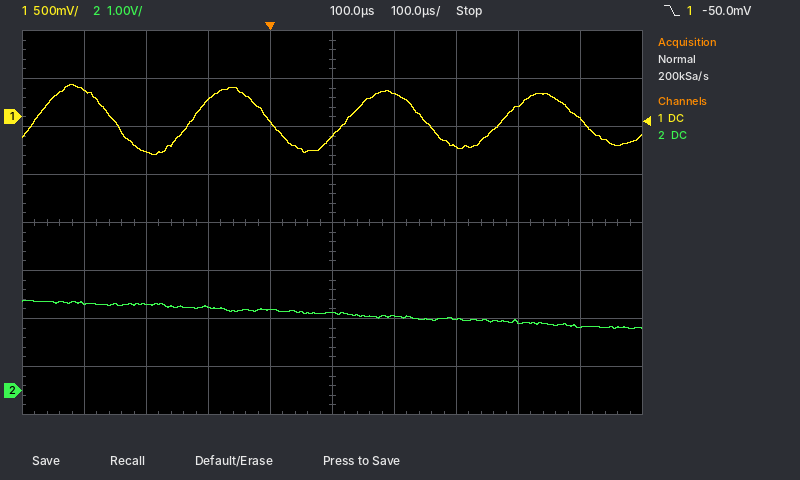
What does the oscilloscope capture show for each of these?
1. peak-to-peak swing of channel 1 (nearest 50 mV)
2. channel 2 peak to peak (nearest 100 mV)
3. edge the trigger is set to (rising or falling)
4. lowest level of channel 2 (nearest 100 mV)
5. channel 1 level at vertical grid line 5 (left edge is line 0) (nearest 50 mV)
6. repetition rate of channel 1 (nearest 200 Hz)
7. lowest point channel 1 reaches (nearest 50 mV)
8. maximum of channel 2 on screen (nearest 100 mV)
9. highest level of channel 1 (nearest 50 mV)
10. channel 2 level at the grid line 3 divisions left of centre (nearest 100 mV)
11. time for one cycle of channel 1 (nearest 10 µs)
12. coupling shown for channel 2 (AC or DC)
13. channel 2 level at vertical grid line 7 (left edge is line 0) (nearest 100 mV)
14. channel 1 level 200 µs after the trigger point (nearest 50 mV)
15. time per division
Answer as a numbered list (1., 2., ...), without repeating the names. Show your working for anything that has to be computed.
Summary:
1. 350 mV − (-400 mV) = 750 mV
2. 1.9 V − (1.3 V) = 600 mV
3. falling
4. 1.3 V
5. -200 mV
6. 1 / 250 µs ≈ 4.0 kHz
7. -400 mV
8. 1.9 V
9. 350 mV
10. 1.8 V
11. 250 µs
12. DC
13. 1.5 V
14. 250 mV
15. 100 µs
